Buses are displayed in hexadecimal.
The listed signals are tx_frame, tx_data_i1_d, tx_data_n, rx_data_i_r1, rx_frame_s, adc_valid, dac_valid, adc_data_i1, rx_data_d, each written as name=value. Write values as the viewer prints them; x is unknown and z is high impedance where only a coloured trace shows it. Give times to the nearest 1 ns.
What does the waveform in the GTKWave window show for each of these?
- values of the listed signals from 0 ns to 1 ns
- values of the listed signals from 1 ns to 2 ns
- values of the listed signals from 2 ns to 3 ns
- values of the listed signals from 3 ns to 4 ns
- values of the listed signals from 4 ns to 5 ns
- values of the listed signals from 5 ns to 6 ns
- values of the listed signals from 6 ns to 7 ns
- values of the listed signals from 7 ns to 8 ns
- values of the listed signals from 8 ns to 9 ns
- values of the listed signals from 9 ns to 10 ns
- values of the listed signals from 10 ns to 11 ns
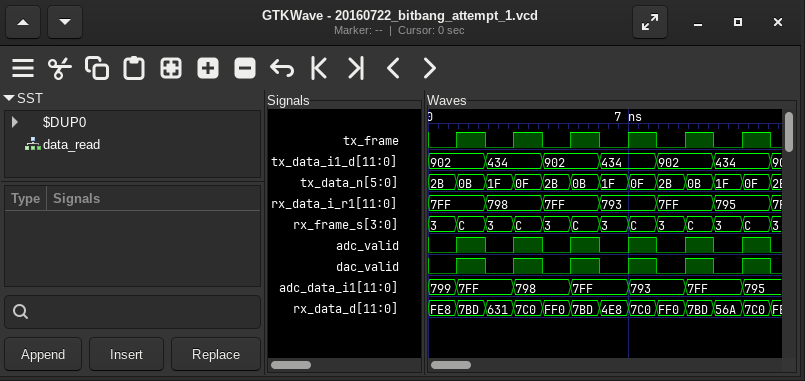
tx_frame=0, tx_data_i1_d=902, tx_data_n=2B, rx_data_i_r1=7FF, rx_frame_s=3, adc_valid=0, dac_valid=0, adc_data_i1=799, rx_data_d=FE8
tx_frame=1, tx_data_i1_d=902, tx_data_n=0B, rx_data_i_r1=7FF, rx_frame_s=C, adc_valid=1, dac_valid=1, adc_data_i1=7FF, rx_data_d=7BD
tx_frame=0, tx_data_i1_d=434, tx_data_n=1F, rx_data_i_r1=798, rx_frame_s=3, adc_valid=0, dac_valid=0, adc_data_i1=7FF, rx_data_d=631
tx_frame=1, tx_data_i1_d=434, tx_data_n=0F, rx_data_i_r1=798, rx_frame_s=C, adc_valid=1, dac_valid=1, adc_data_i1=798, rx_data_d=7C0
tx_frame=0, tx_data_i1_d=902, tx_data_n=2B, rx_data_i_r1=7FF, rx_frame_s=3, adc_valid=0, dac_valid=0, adc_data_i1=798, rx_data_d=FF0
tx_frame=1, tx_data_i1_d=902, tx_data_n=0B, rx_data_i_r1=7FF, rx_frame_s=C, adc_valid=1, dac_valid=1, adc_data_i1=7FF, rx_data_d=7BD
tx_frame=0, tx_data_i1_d=434, tx_data_n=1F, rx_data_i_r1=793, rx_frame_s=3, adc_valid=0, dac_valid=0, adc_data_i1=7FF, rx_data_d=4E8
tx_frame=1, tx_data_i1_d=434, tx_data_n=0F, rx_data_i_r1=793, rx_frame_s=C, adc_valid=1, dac_valid=1, adc_data_i1=793, rx_data_d=7C0
tx_frame=0, tx_data_i1_d=902, tx_data_n=2B, rx_data_i_r1=7FF, rx_frame_s=3, adc_valid=0, dac_valid=0, adc_data_i1=793, rx_data_d=FF0
tx_frame=1, tx_data_i1_d=902, tx_data_n=0B, rx_data_i_r1=7FF, rx_frame_s=C, adc_valid=1, dac_valid=1, adc_data_i1=7FF, rx_data_d=7BD
tx_frame=0, tx_data_i1_d=434, tx_data_n=1F, rx_data_i_r1=795, rx_frame_s=3, adc_valid=0, dac_valid=0, adc_data_i1=7FF, rx_data_d=56A
